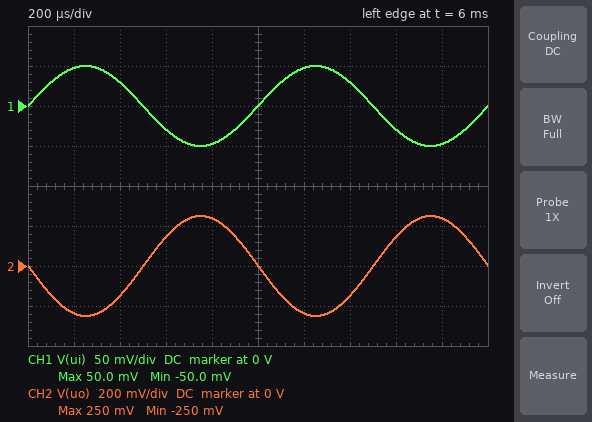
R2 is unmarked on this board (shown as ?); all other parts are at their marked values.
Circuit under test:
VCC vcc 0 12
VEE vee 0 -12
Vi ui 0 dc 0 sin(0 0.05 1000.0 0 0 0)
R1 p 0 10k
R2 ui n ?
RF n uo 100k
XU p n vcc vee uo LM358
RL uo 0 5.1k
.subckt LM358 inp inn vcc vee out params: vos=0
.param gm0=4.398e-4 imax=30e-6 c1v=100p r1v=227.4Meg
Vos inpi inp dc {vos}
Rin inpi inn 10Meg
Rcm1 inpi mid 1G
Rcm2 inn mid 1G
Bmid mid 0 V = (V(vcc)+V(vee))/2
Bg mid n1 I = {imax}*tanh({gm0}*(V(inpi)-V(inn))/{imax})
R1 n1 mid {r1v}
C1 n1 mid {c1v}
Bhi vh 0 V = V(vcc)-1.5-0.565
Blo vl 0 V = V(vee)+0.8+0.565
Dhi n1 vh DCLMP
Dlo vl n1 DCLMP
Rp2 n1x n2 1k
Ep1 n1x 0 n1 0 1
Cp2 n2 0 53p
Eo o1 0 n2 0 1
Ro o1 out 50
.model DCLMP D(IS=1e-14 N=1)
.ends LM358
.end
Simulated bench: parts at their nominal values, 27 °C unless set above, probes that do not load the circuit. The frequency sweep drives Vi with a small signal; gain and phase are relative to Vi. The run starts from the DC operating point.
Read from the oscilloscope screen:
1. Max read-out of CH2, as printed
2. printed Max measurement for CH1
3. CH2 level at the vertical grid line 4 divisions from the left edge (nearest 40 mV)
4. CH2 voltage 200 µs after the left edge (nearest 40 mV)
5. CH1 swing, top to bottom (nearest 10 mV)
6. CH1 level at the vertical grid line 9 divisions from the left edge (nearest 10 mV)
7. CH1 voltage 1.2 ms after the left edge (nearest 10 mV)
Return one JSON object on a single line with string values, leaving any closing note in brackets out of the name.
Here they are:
{"Max read-out of CH2, as printed": "250 mV", "printed Max measurement for CH1": "50.0 mV", "CH2 level at the vertical grid line 4 divisions from the left edge": "240 mV", "CH2 voltage 200 µs after the left edge": "-240 mV", "CH1 swing, top to bottom": "100 mV", "CH1 level at the vertical grid line 9 divisions from the left edge": "-50 mV", "CH1 voltage 1.2 ms after the left edge": "50 mV"}
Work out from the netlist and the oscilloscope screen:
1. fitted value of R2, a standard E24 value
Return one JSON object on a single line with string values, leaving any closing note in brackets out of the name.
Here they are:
{"fitted value of R2, a standard E24 value": "20 kΩ"}
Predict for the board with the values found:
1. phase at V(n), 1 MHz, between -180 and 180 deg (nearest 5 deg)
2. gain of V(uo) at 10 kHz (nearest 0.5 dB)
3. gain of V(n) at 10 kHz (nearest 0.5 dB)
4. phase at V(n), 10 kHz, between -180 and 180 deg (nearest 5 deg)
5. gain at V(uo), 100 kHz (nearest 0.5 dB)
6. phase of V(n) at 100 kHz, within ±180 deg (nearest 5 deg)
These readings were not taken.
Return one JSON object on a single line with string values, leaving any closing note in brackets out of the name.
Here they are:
{"phase at V(n), 1 MHz, between -180 and 180 deg": "5 deg", "gain of V(uo) at 10 kHz": "14.0 dB", "gain of V(n) at 10 kHz": "-23.0 dB", "phase at V(n), 10 kHz, between -180 and 180 deg": "85 deg", "gain at V(uo), 100 kHz": "11.5 dB", "phase of V(n) at 100 kHz, within ±180 deg": "50 deg"}
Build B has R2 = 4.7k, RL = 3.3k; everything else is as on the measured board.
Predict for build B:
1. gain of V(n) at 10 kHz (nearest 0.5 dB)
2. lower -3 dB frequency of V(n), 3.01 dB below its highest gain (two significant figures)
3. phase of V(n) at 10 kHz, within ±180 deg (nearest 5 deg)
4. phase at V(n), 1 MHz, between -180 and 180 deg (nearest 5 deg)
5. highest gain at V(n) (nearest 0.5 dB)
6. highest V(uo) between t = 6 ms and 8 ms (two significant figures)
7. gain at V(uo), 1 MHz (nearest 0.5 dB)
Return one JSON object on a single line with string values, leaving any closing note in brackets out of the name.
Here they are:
{"gain of V(n) at 10 kHz": "-10.5 dB", "lower -3 dB frequency of V(n), 3.01 dB below its highest gain": "31 kHz", "phase of V(n) at 10 kHz, within ±180 deg": "70 deg", "phase at V(n), 1 MHz, between -180 and 180 deg": "0 deg", "highest gain at V(n)": "-0.5 dB", "highest V(uo) between t = 6 ms and 8 ms": "1.1 V", "gain at V(uo), 1 MHz": "-4.0 dB"}
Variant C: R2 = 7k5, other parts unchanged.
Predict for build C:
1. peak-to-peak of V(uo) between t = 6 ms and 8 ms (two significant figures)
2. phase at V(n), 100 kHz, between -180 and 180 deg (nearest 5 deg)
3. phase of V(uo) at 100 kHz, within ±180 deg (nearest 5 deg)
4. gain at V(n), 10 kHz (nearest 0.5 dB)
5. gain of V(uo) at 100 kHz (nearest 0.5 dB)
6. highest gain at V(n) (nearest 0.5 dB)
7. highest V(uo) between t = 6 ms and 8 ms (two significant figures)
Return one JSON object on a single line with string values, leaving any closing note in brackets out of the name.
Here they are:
{"peak-to-peak of V(uo) between t = 6 ms and 8 ms": "1.3 V", "phase at V(n), 100 kHz, between -180 and 180 deg": "25 deg", "phase of V(uo) at 100 kHz, within ±180 deg": "115 deg", "gain at V(n), 10 kHz": "-14.5 dB", "gain of V(uo) at 100 kHz": "15.5 dB", "highest gain at V(n)": "-0.5 dB", "highest V(uo) between t = 6 ms and 8 ms": "670 mV"}
